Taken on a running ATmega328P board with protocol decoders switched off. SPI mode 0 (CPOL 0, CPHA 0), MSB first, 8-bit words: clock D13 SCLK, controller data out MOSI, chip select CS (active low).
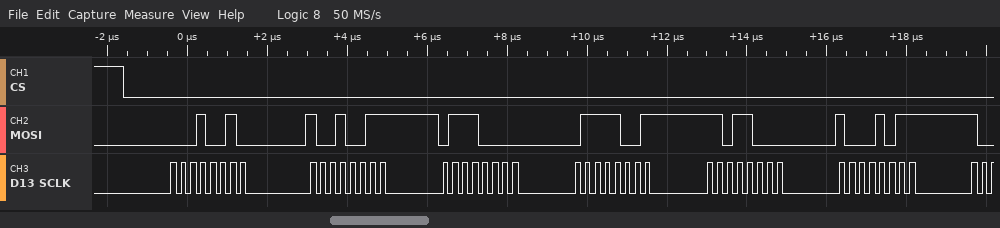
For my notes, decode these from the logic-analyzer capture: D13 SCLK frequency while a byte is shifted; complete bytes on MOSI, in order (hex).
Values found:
4 MHz
12 93 70 79 D8 8B
